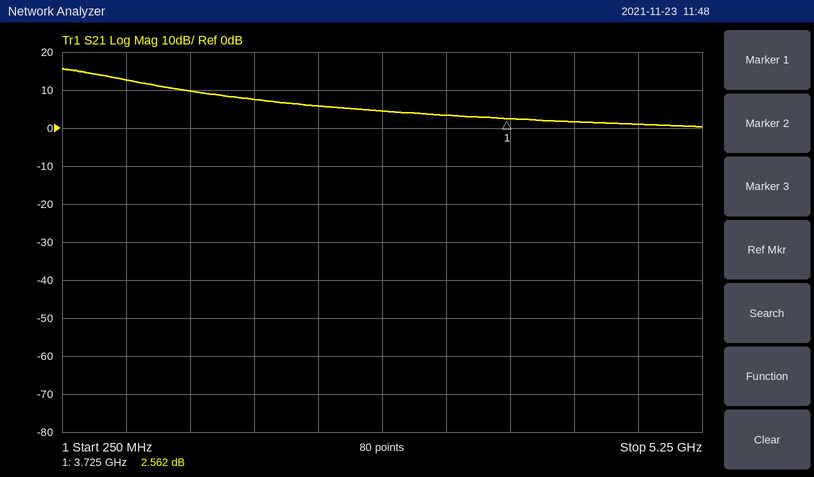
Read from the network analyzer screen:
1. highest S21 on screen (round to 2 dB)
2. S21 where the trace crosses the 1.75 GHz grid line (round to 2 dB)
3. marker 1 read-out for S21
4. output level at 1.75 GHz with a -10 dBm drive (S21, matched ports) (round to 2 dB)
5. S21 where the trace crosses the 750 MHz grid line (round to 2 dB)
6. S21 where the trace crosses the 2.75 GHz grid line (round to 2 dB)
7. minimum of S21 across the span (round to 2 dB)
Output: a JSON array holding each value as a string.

["16 dB", "8 dB", "2.562 dB", "-2 dBm", "12 dB", "4 dB", "0 dB"]
